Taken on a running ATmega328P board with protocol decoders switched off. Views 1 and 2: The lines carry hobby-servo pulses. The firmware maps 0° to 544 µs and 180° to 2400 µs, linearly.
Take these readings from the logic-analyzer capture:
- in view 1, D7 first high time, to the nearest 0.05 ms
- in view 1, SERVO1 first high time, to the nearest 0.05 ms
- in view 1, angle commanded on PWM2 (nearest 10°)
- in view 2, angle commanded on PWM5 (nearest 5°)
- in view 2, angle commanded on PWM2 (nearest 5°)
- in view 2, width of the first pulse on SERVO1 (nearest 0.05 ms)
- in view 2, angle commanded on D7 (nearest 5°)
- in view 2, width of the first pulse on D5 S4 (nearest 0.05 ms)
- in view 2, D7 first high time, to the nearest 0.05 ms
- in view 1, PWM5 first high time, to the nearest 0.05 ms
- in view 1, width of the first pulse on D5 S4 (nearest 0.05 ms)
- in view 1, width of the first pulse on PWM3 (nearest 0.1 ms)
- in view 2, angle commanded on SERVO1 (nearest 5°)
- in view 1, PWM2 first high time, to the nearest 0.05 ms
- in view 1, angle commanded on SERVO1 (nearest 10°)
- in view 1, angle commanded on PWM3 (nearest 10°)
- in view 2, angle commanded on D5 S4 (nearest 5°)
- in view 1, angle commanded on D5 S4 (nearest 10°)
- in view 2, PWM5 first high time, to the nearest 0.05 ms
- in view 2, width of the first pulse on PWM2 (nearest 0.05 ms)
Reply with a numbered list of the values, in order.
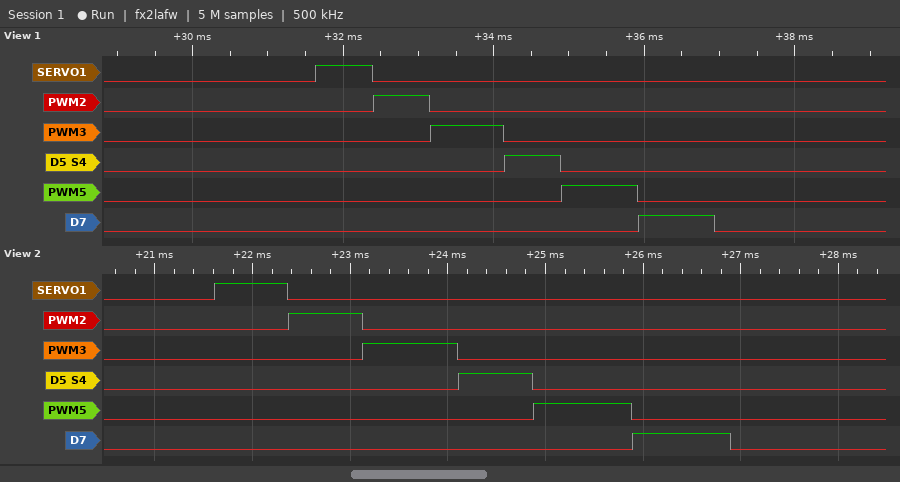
1. 1.00 ms
2. 0.75 ms
3. 20°
4. 45°
5. 20°
6. 0.75 ms
7. 45°
8. 0.75 ms
9. 1.00 ms
10. 1.00 ms
11. 0.75 ms
12. 1.0 ms
13. 20°
14. 0.75 ms
15. 20°
16. 40°
17. 20°
18. 20°
19. 1.00 ms
20. 0.75 ms
